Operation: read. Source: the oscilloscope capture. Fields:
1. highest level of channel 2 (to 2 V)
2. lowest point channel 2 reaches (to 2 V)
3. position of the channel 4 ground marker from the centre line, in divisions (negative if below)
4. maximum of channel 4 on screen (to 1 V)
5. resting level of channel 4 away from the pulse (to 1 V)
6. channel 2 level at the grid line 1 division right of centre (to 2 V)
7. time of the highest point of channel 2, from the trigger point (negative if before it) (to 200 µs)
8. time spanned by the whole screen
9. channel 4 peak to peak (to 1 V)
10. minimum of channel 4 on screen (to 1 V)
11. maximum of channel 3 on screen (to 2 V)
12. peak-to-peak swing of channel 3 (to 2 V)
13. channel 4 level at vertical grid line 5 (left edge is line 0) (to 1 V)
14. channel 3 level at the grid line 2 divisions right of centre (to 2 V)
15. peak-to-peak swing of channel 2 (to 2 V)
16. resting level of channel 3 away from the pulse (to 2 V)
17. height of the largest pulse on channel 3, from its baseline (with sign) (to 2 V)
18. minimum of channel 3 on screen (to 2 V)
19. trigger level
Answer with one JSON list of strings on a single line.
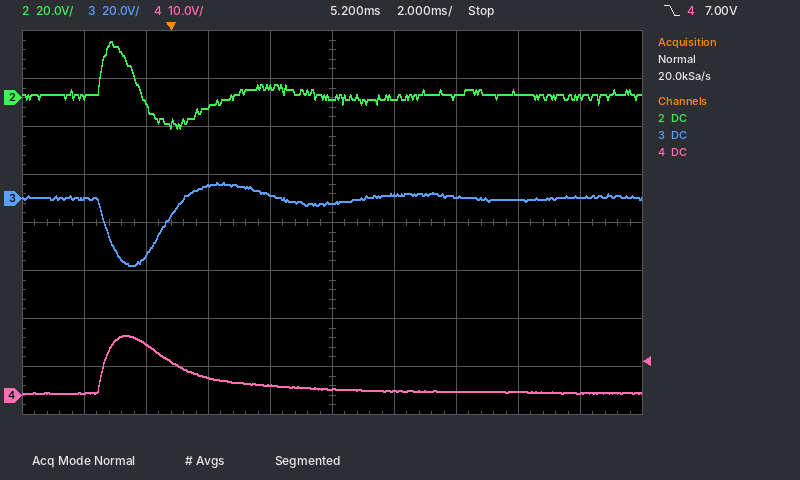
["24 V", "-12 V", "-3.6 div", "12 V", "1 V", "0 V", "-2.0 ms", "20 ms", "12 V", "0 V", "6 V", "34 V", "1 V", "0 V", "36 V", "0 V", "-28 V", "-28 V", "7.00 V"]
